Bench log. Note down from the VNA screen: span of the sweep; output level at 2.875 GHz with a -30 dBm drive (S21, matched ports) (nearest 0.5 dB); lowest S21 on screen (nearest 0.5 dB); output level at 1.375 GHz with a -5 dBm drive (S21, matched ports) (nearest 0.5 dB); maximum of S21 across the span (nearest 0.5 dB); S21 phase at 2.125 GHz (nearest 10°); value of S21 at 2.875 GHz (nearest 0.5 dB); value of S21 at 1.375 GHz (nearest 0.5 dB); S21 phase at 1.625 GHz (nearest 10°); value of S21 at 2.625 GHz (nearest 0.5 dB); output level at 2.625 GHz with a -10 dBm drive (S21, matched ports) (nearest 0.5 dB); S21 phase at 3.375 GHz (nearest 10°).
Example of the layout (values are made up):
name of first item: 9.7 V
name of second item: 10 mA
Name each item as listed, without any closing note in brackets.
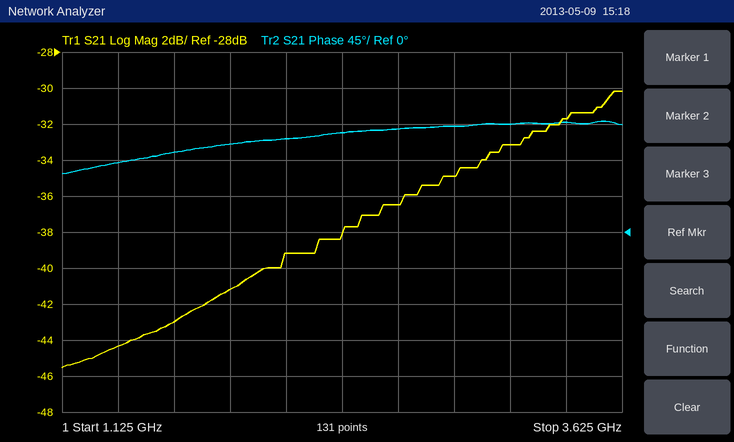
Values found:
span of the sweep: 2.5 GHz
output level at 2.875 GHz with a -30 dBm drive (S21, matched ports): -65.0 dBm
lowest S21 on screen: -45.5 dB
output level at 1.375 GHz with a -5 dBm drive (S21, matched ports): -49.5 dBm
maximum of S21 across the span: -30.0 dB
S21 phase at 2.125 GHz: 120°
value of S21 at 2.875 GHz: -35.0 dB
value of S21 at 1.375 GHz: -44.5 dB
S21 phase at 1.625 GHz: 100°
value of S21 at 2.625 GHz: -36.5 dB
output level at 2.625 GHz with a -10 dBm drive (S21, matched ports): -46.5 dBm
S21 phase at 3.375 GHz: 140°
